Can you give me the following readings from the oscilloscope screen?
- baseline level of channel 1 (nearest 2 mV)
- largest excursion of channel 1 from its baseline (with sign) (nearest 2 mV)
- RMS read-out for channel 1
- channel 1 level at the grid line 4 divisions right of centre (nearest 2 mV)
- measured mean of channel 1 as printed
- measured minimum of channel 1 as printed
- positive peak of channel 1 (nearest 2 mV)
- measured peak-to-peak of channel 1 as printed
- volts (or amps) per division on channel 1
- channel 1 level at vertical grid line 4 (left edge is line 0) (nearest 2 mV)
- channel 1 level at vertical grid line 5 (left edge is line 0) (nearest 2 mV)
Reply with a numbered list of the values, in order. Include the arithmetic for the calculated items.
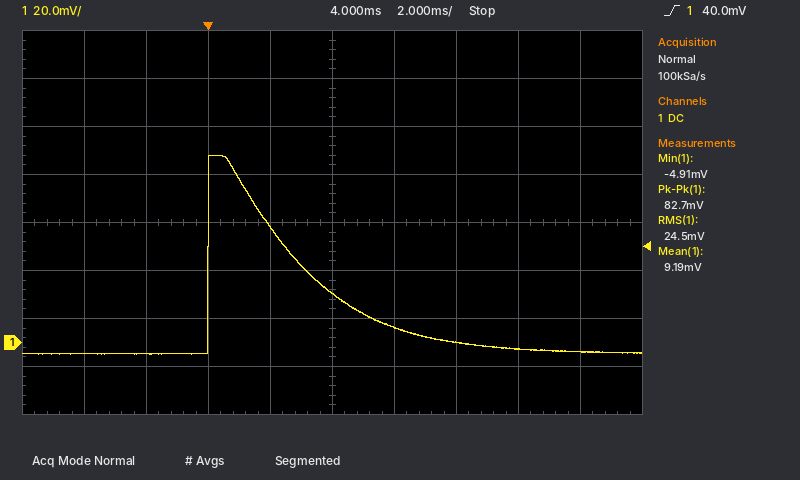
1. -4 mV
2. 78 mV − (-4 mV) = +82 mV
3. 24.5 mV
4. -4 mV
5. 9.19 mV
6. -4.91 mV
7. 78 mV
8. 82.7 mV
9. 20 mV
10. 48 mV
11. 20 mV
